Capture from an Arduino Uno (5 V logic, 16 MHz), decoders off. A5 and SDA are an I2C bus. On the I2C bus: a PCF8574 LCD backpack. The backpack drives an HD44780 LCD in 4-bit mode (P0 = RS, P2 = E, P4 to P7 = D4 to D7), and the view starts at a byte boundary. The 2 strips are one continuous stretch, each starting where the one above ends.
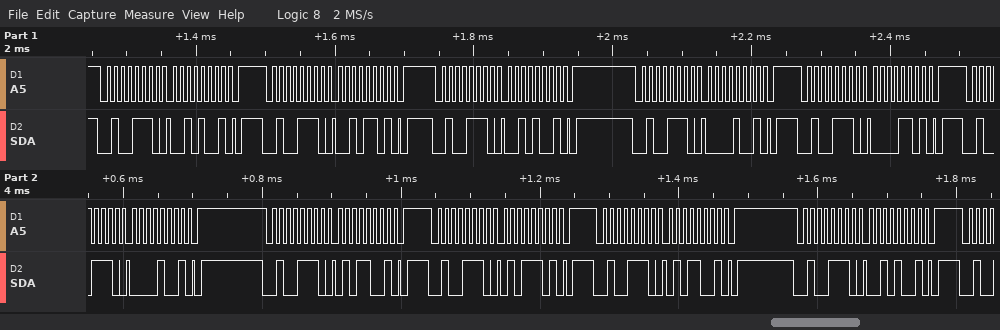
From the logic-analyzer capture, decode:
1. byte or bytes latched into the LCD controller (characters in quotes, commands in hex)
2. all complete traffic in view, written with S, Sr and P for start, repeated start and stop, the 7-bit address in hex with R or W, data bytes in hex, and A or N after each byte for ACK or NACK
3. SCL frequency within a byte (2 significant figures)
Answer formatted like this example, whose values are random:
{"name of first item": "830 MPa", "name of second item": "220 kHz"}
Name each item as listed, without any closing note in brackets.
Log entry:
{"byte or bytes latched into the LCD controller": "' '", "all complete traffic in view, written with S, Sr and P for start, repeated start and stop, the 7-bit address in hex with R or W, data bytes in hex, and A or N after each byte for ACK or NACK": "S 27W A 29 A P S 27W A 2D A P S 27W A 29 A P S 27W A 09 A P S 27W A 0D A P S 27W A 09 A P S 27W A 59 A P S 27W A 5D A P S 27W A 59 A P S 27W A 29 A P", "SCL frequency within a byte": "100 kHz"}
